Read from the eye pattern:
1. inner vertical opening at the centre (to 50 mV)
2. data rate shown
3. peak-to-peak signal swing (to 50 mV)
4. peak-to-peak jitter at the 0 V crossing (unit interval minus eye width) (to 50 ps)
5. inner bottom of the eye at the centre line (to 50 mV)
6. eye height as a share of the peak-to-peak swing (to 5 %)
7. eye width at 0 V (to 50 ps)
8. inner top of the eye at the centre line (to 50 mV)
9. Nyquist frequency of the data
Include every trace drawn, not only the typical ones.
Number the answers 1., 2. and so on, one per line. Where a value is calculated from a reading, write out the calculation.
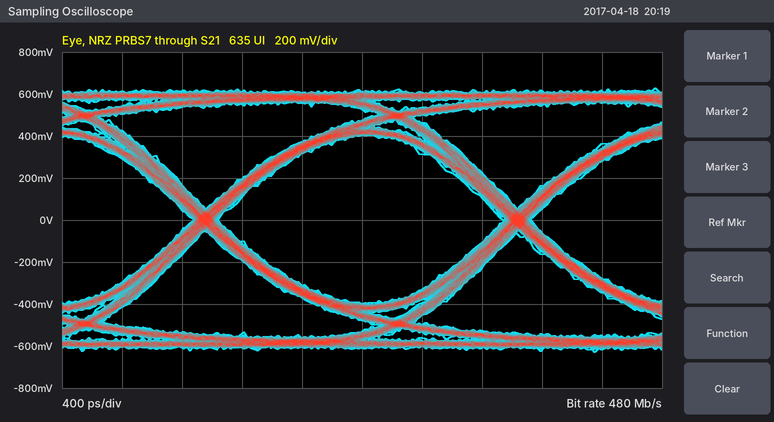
1. 800 mV
2. 480 Mb/s
3. 1.25 V
4. 200 ps
5. -400 mV
6. 800 mV / 1.25 V ≈ 64.0 %, so 65 % to the nearest 5 %
7. 1.90 ns
8. 400 mV
9. 240 MHz
